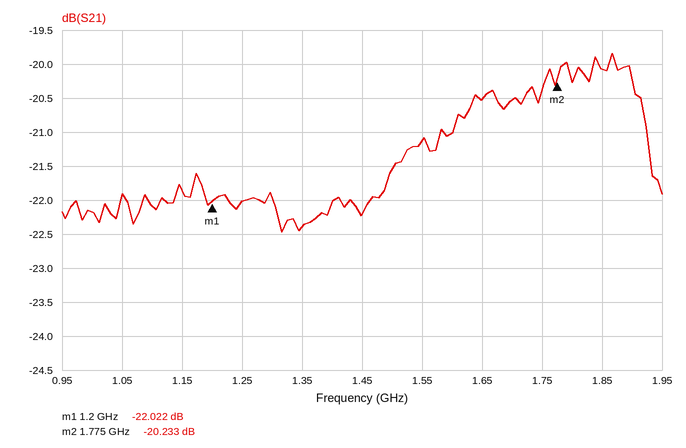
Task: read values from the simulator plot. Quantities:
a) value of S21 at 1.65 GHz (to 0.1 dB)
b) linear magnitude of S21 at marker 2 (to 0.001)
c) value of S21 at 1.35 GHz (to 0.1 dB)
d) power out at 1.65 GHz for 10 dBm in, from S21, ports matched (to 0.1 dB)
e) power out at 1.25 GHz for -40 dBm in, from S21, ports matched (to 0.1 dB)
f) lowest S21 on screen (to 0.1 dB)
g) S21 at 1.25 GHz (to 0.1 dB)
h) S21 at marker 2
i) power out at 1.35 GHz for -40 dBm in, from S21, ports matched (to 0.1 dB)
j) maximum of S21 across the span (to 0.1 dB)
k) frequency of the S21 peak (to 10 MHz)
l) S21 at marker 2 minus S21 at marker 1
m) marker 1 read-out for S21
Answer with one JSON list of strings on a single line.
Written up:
["-20.5 dB", "0.097", "-22.4 dB", "-10.5 dBm", "-62.0 dBm", "-22.5 dB", "-22.0 dB", "-20.233 dB", "-62.4 dBm", "-19.8 dB", "1.87 GHz", "1.789 dB", "-22.022 dB"]
